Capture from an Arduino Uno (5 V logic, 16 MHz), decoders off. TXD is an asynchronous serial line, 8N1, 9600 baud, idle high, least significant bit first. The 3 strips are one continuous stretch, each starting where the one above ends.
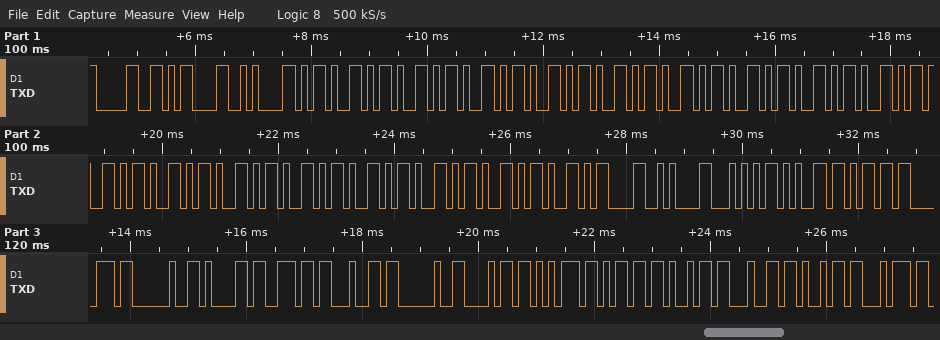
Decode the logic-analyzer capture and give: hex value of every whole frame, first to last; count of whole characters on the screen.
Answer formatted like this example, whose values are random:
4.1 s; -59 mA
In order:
0x30 0x0D 0x0A 0x2D 0x2D 0x2D 0x2D 0x2D 0x2D 0x2D 0x2D 0x2D 0x2D 0x2D 0x2D 0x2D 0x2D 0x2D 0x2D 0x2D 0x0D 0x0A 0x54 0x65 0x6D 0x70 0x20 0x61 0x6E 0x64 0x20 0x68 0x75 0x6D 0x69 0x64 0x69 0x74; 38
